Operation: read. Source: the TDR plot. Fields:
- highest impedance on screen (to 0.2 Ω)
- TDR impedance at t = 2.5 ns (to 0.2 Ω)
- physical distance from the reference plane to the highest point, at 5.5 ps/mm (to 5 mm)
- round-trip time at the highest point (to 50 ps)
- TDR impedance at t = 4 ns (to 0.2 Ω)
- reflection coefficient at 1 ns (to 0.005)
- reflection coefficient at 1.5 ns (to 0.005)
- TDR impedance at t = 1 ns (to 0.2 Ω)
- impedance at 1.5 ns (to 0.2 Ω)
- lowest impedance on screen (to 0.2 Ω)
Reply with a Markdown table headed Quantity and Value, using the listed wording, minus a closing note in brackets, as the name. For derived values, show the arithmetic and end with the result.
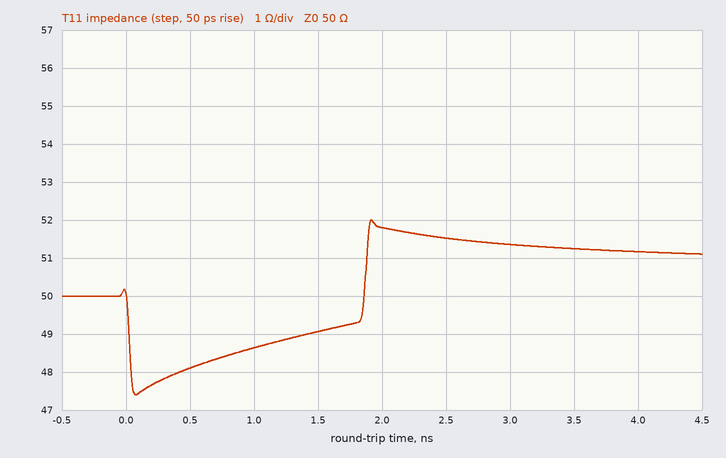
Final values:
| Quantity | Value |
|---|---|
| highest impedance on screen | 52.0 Ω |
| TDR impedance at t = 2.5 ns | 51.6 Ω |
| physical distance from the reference plane to the highest point, at 5.5 ps/mm | 1.90 ns / 2 / 5.5 ps/mm ≈ 173 mm, so 175 mm to the nearest 5 mm |
| round-trip time at the highest point | 1.90 ns |
| TDR impedance at t = 4 ns | 51.2 Ω |
| reflection coefficient at 1 ns | (48.6 − 50)/(48.6 + 50) ≈ -0.0142, so -0.015 to the nearest 0.005 |
| reflection coefficient at 1.5 ns | (49 − 50)/(49 + 50) ≈ -0.010 |
| TDR impedance at t = 1 ns | 48.6 Ω |
| impedance at 1.5 ns | 49.0 Ω |
| lowest impedance on screen | 47.4 Ω |
